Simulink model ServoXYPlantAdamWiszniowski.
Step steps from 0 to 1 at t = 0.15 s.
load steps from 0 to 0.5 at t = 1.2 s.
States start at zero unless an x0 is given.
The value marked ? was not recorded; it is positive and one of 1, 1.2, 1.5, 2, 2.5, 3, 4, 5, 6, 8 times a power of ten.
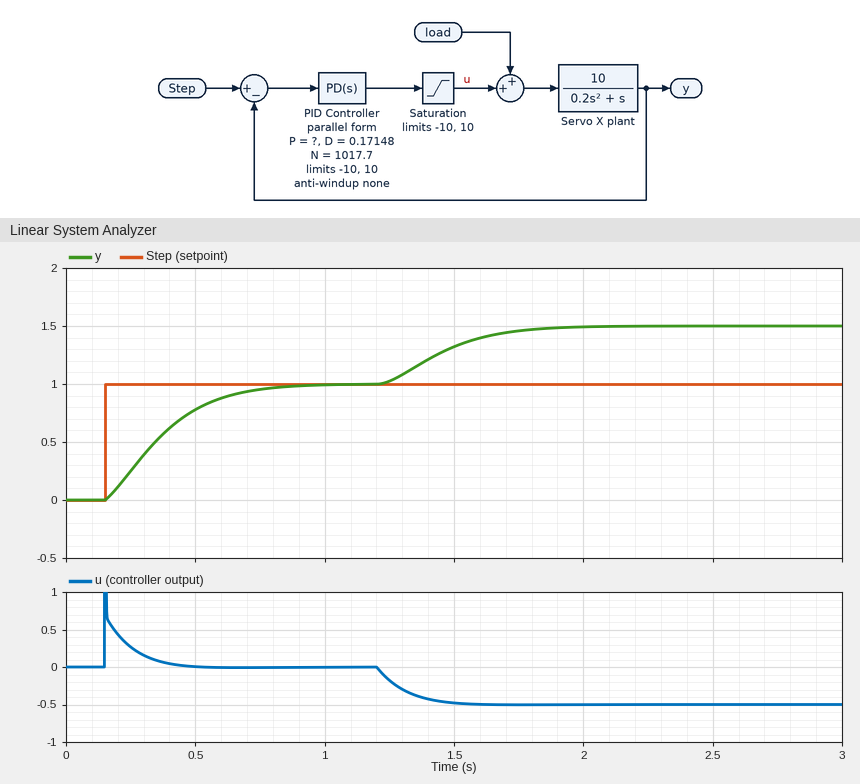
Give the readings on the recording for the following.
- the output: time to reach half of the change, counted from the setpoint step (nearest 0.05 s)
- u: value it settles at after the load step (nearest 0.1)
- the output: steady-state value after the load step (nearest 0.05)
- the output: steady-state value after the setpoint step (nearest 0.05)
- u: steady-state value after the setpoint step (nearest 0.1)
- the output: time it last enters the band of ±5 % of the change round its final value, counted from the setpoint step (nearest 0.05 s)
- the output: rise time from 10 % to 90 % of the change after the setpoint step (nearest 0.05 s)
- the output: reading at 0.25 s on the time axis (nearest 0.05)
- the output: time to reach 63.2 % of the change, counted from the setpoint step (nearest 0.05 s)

0.20 s
-0.5
1.50
1.00
0.0
0.60 s
0.45 s
0.25
0.25 s
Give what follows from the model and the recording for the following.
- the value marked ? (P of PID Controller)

1
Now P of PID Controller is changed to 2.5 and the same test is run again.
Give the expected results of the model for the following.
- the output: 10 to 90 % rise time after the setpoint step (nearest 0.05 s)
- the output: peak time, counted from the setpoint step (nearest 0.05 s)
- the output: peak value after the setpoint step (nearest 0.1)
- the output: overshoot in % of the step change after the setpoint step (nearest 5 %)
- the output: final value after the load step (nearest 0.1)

0.15 s
0.35 s
1.1
10 %
1.2
